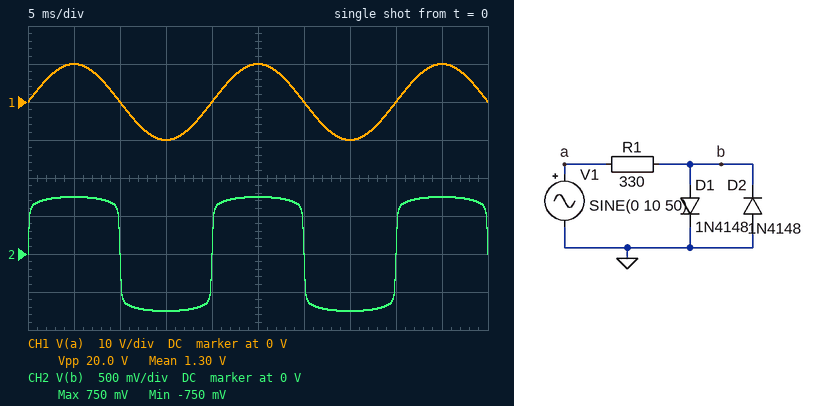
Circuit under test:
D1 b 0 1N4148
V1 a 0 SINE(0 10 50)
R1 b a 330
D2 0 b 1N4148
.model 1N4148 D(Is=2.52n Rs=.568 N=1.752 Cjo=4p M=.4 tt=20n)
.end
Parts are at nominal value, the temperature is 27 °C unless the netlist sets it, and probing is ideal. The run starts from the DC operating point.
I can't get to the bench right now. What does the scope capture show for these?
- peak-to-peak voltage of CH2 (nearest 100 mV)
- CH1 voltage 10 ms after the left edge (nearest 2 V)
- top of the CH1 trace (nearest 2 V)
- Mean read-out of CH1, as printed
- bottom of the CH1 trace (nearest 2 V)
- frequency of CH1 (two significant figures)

1.5 V
0 V
10 V
1.30 V
-10 V
50 Hz
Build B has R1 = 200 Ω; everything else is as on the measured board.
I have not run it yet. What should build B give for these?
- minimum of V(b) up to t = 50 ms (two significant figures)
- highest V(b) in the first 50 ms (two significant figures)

-780 mV
780 mV
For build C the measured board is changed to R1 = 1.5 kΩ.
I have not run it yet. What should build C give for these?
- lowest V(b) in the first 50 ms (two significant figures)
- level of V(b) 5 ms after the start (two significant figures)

-670 mV
670 mV
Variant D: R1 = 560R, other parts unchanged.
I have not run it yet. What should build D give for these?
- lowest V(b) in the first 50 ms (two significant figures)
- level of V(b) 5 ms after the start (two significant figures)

-720 mV
720 mV
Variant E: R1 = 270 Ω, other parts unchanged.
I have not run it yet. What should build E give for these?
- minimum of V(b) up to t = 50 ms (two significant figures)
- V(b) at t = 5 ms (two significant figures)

-760 mV
760 mV
